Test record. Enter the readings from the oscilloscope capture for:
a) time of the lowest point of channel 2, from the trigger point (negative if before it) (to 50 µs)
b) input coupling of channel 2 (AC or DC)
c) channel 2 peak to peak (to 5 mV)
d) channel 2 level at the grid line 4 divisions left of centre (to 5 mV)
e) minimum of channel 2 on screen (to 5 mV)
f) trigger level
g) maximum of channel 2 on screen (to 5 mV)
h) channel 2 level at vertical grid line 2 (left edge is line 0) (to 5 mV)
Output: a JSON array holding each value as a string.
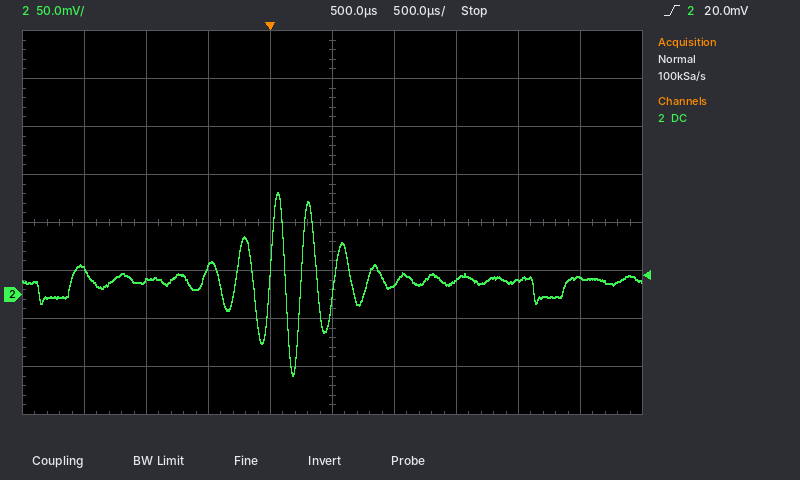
["+200 µs", "DC", "190 mV", "25 mV", "-85 mV", "20.0 mV", "105 mV", "15 mV"]
